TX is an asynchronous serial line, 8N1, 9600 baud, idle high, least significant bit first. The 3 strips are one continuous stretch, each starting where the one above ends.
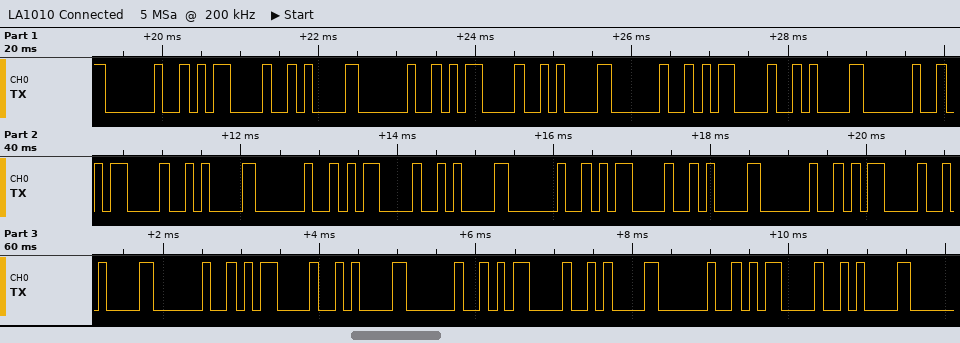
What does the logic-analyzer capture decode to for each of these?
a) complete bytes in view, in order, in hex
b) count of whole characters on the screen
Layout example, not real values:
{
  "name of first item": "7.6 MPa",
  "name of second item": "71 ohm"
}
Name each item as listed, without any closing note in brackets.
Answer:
{
  "complete bytes in view, in order, in hex": "0x20 0x0D 0x0A 0x20 0x0D 0x0A 0x20 0x0D 0x0A 0x20 0x0D 0x0A 0x20 0x0D 0x0A 0x20 0x0D 0x0A 0x20 0x0D 0x0A 0x20 0x0D 0x0A 0x20 0x0D 0x0A 0x20 0x0D 0x0A",
  "count of whole characters on the screen": "30"
}
